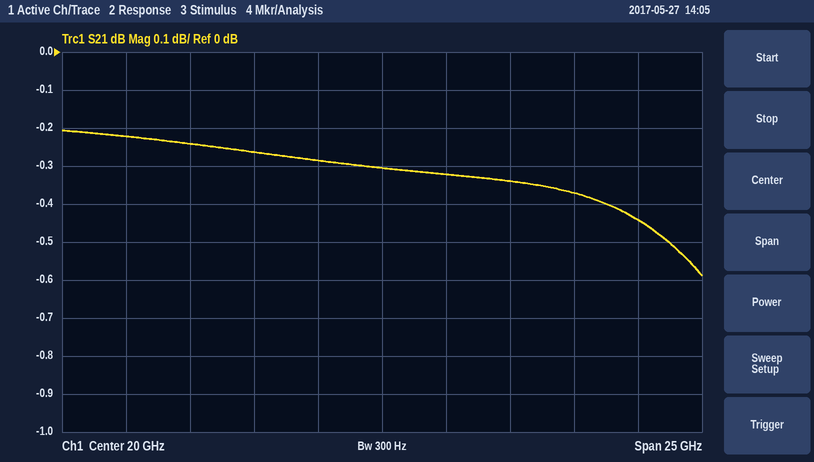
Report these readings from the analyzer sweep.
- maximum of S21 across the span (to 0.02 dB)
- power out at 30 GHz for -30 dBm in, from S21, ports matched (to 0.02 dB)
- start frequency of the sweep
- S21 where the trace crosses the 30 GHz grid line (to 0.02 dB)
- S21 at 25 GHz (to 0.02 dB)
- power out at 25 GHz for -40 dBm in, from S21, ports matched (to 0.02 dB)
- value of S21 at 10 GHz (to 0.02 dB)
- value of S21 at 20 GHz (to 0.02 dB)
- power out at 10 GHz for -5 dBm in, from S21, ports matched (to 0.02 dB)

-0.20 dB
-30.44 dBm
7.5 GHz
-0.44 dB
-0.34 dB
-40.34 dBm
-0.22 dB
-0.30 dB
-5.22 dBm
